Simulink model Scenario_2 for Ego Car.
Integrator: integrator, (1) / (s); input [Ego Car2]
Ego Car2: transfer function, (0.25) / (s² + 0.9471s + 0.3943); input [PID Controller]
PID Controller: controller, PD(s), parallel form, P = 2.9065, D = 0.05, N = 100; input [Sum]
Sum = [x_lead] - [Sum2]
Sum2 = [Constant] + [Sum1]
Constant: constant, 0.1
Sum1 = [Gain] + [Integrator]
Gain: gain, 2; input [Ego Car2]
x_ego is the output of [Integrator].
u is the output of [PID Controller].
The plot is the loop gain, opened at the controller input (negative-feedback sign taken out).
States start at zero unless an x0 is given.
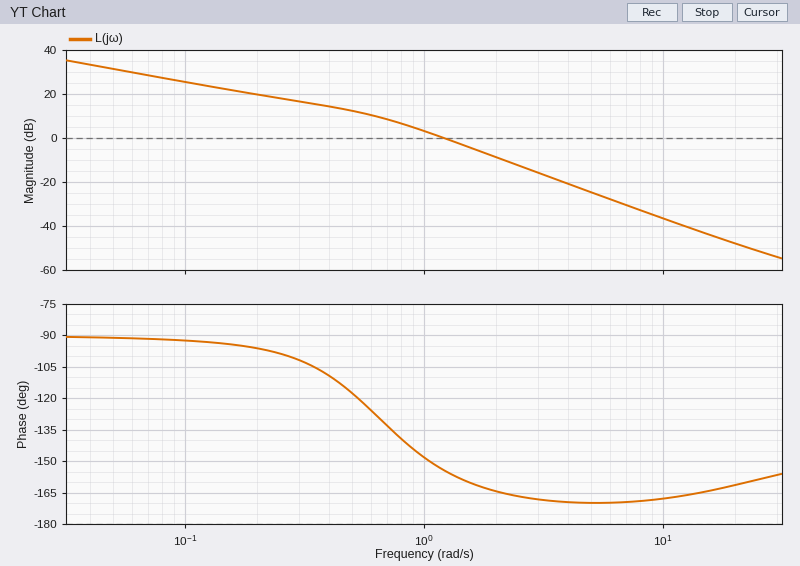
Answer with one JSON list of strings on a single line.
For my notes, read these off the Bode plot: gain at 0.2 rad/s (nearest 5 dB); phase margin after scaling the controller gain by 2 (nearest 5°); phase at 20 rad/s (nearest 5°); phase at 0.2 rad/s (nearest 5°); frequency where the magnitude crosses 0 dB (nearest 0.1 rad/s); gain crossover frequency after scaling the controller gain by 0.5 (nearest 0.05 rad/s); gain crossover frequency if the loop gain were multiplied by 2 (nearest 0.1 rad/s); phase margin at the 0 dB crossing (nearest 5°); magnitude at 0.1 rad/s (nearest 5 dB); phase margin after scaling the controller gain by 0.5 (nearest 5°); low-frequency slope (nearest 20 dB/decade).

["20 dB", "20°", "-160°", "-95°", "1.2 rad/s", "0.85 rad/s", "1.7 rad/s", "25°", "25 dB", "40°", "-20 dB/decade"]
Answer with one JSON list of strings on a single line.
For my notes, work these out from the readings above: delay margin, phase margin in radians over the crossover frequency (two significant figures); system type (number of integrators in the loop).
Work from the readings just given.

["0.36 s", "1"]
